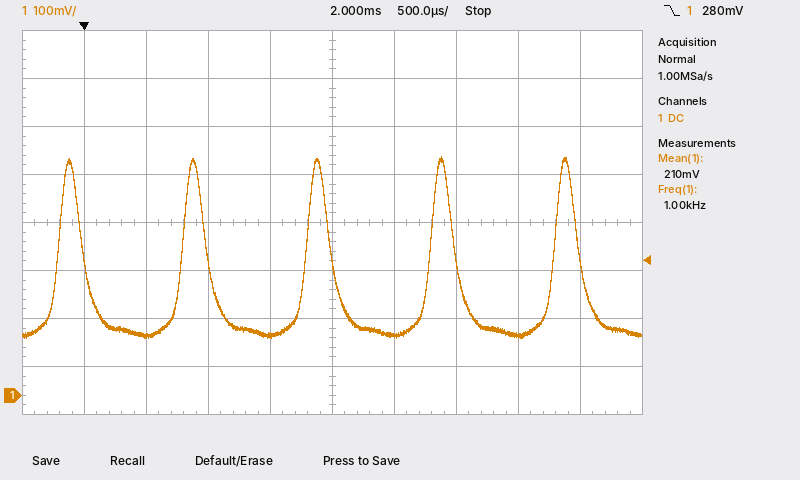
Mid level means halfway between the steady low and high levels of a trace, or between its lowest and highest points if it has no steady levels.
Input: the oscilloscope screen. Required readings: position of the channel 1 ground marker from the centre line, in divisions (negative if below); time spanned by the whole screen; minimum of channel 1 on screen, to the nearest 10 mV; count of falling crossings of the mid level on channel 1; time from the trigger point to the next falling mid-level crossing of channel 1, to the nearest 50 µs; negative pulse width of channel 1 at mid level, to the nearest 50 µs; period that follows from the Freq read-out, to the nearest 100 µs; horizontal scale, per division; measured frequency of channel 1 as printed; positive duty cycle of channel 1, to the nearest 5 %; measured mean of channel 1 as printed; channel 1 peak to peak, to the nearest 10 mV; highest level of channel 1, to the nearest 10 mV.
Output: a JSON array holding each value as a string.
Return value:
["-3.6 div", "5 ms", "120 mV", "5", "1.00 ms", "800 µs", "1.0 ms", "500 µs", "1.00 kHz", "20 %", "210 mV", "380 mV", "500 mV"]
